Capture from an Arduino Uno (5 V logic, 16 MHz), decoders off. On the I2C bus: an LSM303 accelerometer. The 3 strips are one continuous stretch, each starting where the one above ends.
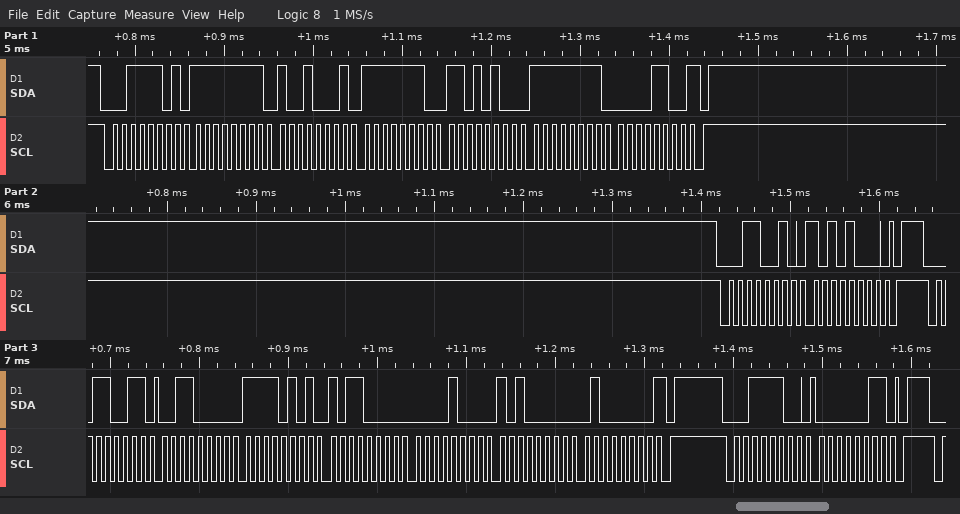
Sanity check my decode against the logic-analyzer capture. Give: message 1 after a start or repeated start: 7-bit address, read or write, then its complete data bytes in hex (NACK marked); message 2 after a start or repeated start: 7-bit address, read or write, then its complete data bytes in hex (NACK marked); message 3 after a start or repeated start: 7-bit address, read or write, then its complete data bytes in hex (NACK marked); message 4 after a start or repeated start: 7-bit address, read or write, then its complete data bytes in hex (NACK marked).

0x1E read: FF 91 FE D4 FF 0C NACK
0x19 write: A8
0x19 read: 30 F5 B0 08 A0 40 NACK
0x1E write: 03
